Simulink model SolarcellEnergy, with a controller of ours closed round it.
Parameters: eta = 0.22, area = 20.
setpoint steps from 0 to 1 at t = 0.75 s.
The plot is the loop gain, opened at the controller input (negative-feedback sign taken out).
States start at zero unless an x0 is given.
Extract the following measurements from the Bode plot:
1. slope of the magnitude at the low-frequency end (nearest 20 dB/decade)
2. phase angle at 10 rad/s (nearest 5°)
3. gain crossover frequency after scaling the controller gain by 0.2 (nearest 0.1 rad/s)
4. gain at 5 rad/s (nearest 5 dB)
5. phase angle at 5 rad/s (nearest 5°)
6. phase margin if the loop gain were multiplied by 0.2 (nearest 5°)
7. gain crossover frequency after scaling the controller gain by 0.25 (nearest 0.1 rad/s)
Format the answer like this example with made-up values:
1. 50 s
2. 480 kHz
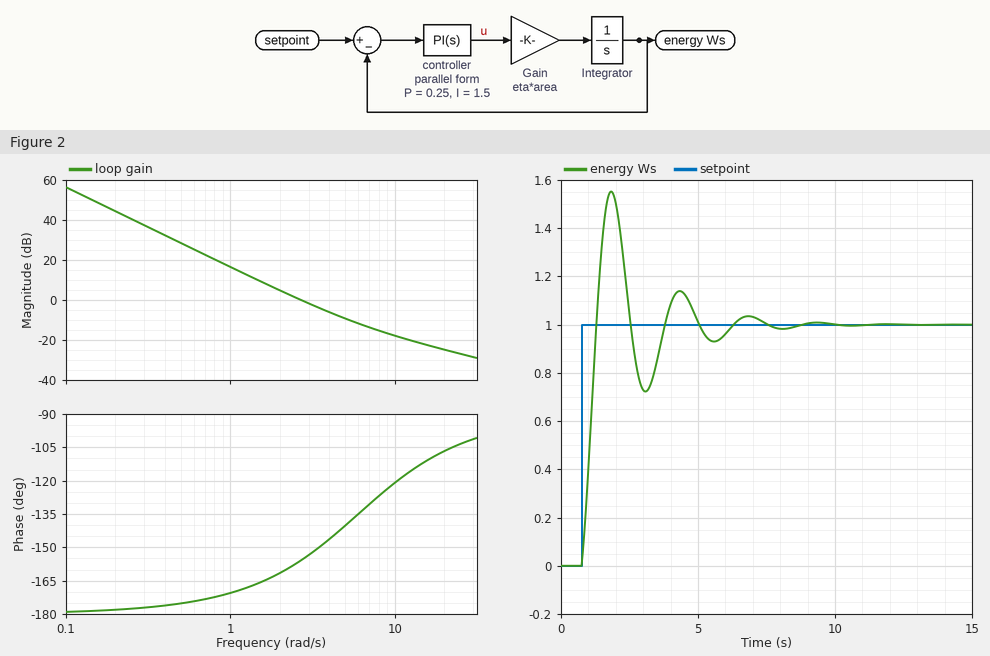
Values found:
1. -40 dB/decade
2. -120°
3. 1.2 rad/s
4. -10 dB
5. -140°
6. 10°
7. 1.3 rad/s
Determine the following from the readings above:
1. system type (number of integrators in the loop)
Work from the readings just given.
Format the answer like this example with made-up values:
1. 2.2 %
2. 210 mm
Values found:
1. 2
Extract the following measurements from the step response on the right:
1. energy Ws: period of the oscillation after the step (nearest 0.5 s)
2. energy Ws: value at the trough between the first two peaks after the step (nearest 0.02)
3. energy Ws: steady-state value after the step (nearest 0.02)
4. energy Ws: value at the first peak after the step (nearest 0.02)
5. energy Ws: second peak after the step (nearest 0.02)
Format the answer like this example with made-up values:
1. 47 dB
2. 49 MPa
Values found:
1. 2.5 s
2. 0.72
3. 1.00
4. 1.56
5. 1.14
